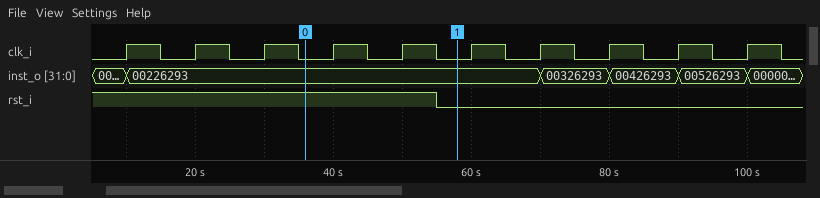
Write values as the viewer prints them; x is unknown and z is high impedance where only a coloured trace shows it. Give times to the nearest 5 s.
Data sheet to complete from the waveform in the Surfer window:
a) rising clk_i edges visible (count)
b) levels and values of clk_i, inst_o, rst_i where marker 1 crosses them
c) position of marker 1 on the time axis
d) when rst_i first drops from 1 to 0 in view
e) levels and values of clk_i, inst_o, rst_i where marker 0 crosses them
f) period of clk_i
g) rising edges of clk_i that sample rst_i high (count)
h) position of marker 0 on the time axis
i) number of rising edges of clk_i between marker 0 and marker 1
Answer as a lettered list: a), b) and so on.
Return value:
a) 10
b) clk_i=0, inst_o=00226293, rst_i=0
c) 60 s
d) 55 s
e) clk_i=0, inst_o=00226293, rst_i=1
f) 10 s
g) 5
h) 35 s
i) 2
